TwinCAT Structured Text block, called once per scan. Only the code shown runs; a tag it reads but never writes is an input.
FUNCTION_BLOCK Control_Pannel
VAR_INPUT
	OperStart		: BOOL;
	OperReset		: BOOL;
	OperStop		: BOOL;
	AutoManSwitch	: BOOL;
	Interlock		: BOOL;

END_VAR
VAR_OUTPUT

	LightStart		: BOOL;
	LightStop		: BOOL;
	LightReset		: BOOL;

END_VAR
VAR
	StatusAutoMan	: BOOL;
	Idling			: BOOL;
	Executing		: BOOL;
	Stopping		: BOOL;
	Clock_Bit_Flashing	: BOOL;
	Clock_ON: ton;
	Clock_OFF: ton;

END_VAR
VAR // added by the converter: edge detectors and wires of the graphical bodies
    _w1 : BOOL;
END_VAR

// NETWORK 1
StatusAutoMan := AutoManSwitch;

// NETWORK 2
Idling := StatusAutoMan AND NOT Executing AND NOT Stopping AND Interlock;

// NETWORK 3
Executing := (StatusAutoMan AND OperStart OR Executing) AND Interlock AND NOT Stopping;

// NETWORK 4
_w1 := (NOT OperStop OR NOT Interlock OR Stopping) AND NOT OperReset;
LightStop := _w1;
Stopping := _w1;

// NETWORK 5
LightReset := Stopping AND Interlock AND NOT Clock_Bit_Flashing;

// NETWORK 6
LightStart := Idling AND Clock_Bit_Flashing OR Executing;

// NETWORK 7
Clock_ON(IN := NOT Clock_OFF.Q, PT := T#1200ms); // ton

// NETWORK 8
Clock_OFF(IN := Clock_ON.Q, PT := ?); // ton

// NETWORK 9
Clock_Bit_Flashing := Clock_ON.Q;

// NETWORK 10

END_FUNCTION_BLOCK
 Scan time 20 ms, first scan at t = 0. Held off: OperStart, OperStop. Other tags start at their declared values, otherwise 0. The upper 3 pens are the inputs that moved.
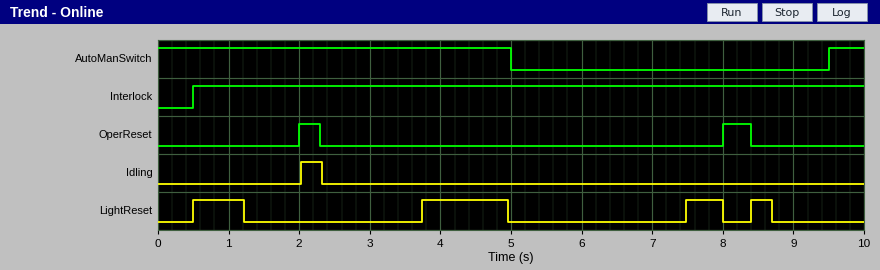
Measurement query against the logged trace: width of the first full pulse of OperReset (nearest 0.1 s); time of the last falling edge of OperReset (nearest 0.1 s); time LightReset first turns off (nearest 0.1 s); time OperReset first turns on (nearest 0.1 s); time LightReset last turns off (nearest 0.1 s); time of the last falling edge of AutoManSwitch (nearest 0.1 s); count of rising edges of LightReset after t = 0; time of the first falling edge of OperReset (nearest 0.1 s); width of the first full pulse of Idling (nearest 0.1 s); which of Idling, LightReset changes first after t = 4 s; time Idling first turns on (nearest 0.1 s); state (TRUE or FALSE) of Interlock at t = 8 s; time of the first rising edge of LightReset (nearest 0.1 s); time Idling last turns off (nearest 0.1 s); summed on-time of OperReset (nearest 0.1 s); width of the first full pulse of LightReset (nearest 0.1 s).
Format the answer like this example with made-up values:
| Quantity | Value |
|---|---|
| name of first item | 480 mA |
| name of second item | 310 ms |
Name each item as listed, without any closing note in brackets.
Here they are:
| Quantity | Value |
|---|---|
| width of the first full pulse of OperReset | 0.3 s |
| time of the last falling edge of OperReset | 8.4 s |
| time LightReset first turns off | 1.2 s |
| time OperReset first turns on | 2.0 s |
| time LightReset last turns off | 8.7 s |
| time of the last falling edge of AutoManSwitch | 5.0 s |
| count of rising edges of LightReset after t = 0 | 4 |
| time of the first falling edge of OperReset | 2.3 s |
| width of the first full pulse of Idling | 0.3 s |
| which of Idling, LightReset changes first after t = 4 s | LightReset |
| time Idling first turns on | 2.0 s |
| state (TRUE or FALSE) of Interlock at t = 8 s | TRUE |
| time of the first rising edge of LightReset | 0.5 s |
| time Idling last turns off | 2.3 s |
| summed on-time of OperReset | 0.7 s |
| width of the first full pulse of LightReset | 0.7 s |
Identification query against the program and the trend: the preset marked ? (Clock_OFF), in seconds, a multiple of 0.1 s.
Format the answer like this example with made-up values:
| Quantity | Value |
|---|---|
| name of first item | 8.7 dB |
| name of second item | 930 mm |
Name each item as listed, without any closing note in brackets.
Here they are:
| Quantity | Value |
|---|---|
| the preset marked ? (Clock_OFF), in seconds, a multiple of 0.1 s | 2.5 s |
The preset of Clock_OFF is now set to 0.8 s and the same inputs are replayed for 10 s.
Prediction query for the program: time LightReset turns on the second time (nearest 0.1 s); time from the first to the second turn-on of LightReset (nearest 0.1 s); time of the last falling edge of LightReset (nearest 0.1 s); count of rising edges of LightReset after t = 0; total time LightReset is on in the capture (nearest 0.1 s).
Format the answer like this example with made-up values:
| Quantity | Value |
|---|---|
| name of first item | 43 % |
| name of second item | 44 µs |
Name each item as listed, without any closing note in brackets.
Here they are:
| Quantity | Value |
|---|---|
| time LightReset turns on the second time | 2.3 s |
| time from the first to the second turn-on of LightReset | 1.8 s |
| time of the last falling edge of LightReset | 9.4 s |
| count of rising edges of LightReset after t = 0 | 5 |
| total time LightReset is on in the capture | 5.1 s |
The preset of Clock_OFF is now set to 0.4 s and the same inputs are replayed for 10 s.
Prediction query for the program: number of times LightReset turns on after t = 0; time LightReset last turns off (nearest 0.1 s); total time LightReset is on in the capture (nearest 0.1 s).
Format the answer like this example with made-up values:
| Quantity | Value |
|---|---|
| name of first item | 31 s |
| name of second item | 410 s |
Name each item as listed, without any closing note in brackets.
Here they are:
| Quantity | Value |
|---|---|
| number of times LightReset turns on after t = 0 | 8 |
| time LightReset last turns off | 9.4 s |
| total time LightReset is on in the capture | 6.5 s |
